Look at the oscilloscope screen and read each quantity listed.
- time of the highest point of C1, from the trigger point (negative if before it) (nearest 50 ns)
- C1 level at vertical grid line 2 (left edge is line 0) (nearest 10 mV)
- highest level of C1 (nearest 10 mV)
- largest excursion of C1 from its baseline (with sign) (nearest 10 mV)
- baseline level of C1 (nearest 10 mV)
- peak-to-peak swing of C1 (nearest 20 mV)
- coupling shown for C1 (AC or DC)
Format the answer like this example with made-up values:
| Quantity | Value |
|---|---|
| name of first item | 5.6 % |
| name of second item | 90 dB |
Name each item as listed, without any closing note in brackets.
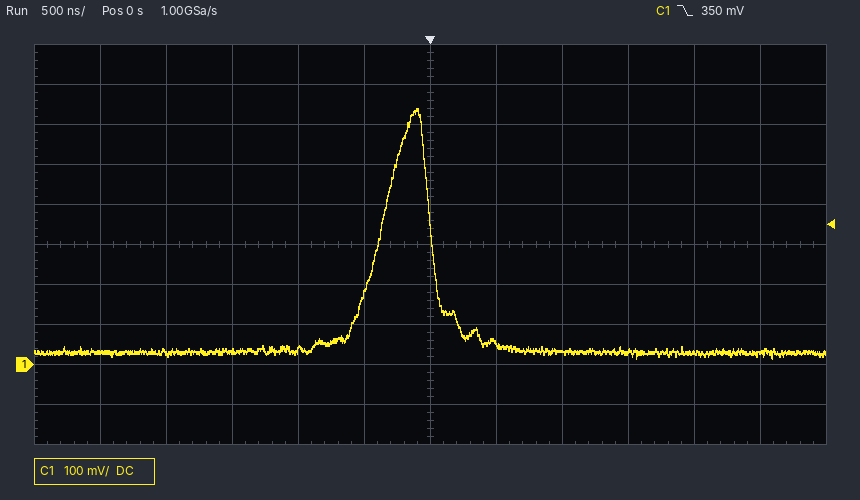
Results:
| Quantity | Value |
|---|---|
| time of the highest point of C1, from the trigger point (negative if before it) | -100 ns |
| C1 level at vertical grid line 2 (left edge is line 0) | 30 mV |
| highest level of C1 | 640 mV |
| largest excursion of C1 from its baseline (with sign) | +610 mV |
| baseline level of C1 | 30 mV |
| peak-to-peak swing of C1 | 620 mV |
| coupling shown for C1 | DC |
